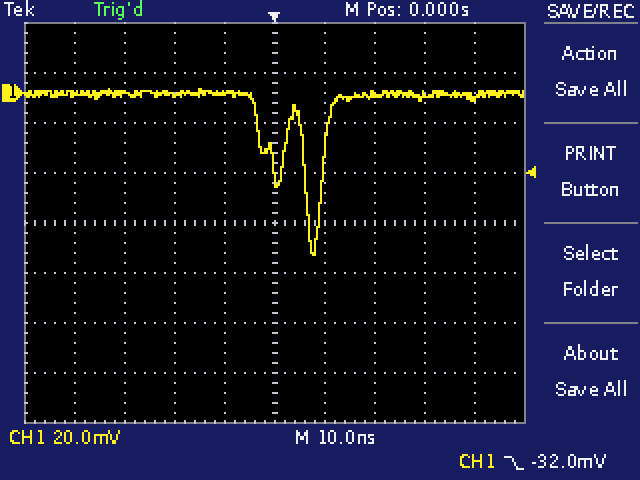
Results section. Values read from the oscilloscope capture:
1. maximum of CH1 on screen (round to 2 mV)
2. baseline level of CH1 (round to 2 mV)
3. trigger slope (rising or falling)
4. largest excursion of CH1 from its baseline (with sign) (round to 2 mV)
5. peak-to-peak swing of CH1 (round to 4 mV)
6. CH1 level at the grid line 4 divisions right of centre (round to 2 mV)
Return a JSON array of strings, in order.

["2 mV", "0 mV", "falling", "-64 mV", "68 mV", "-2 mV"]
